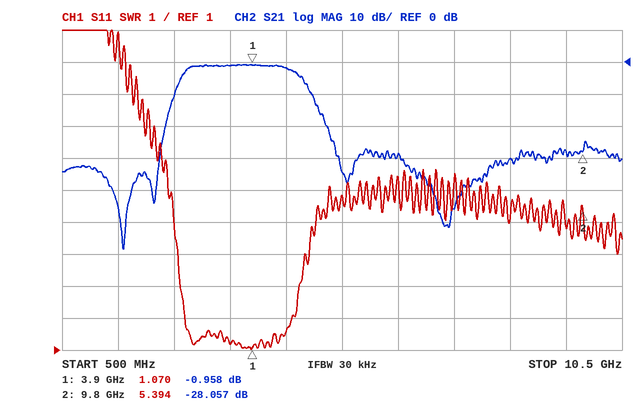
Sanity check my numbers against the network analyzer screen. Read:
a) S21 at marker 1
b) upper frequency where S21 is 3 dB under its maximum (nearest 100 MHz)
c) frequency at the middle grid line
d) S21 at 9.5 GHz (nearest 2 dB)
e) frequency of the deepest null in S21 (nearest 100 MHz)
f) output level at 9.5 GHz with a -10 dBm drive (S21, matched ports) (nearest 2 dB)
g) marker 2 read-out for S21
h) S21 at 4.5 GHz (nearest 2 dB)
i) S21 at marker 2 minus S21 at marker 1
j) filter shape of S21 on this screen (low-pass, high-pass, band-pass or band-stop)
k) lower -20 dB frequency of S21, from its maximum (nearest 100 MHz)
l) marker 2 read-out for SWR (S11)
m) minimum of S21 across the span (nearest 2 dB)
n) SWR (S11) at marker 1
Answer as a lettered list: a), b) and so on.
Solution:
a) -0.958 dB
b) 4.7 GHz
c) 5.5 GHz
d) -28 dB
e) 1.6 GHz
f) -38 dBm
g) -28.057 dB
h) -2 dB
i) -27.099 dB
j) band-pass
k) 2.3 GHz
l) 5.394
m) -58 dB
n) 1.070
